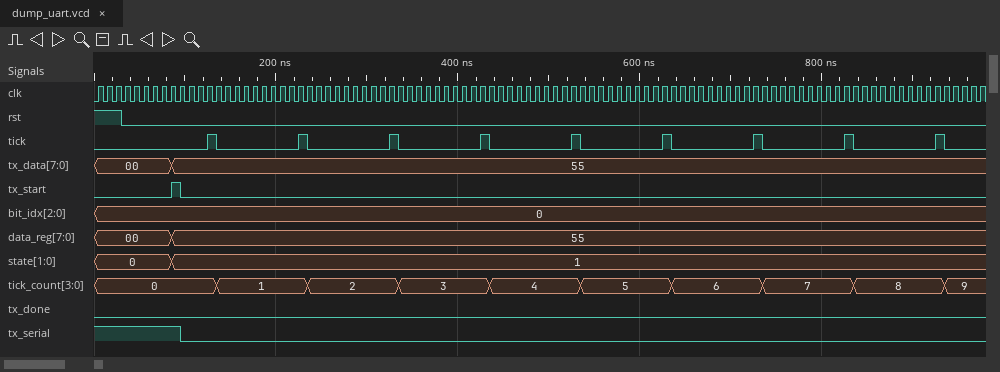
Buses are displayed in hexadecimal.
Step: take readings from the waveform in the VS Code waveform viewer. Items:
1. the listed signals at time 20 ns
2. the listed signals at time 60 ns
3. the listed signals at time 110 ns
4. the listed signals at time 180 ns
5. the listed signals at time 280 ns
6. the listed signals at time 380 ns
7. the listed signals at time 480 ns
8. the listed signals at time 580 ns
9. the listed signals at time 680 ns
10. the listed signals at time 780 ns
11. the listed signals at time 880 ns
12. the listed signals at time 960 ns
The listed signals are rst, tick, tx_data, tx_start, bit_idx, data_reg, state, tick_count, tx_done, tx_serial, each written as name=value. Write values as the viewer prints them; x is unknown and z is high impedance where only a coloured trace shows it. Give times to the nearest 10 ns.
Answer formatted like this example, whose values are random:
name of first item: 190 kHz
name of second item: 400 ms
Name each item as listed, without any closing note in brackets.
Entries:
the listed signals at time 20 ns: rst=1, tick=0, tx_data=00, tx_start=0, bit_idx=0, data_reg=00, state=0, tick_count=0, tx_done=0, tx_serial=1
the listed signals at time 60 ns: rst=0, tick=0, tx_data=00, tx_start=0, bit_idx=0, data_reg=00, state=0, tick_count=0, tx_done=0, tx_serial=1
the listed signals at time 110 ns: rst=0, tick=0, tx_data=55, tx_start=0, bit_idx=0, data_reg=55, state=1, tick_count=0, tx_done=0, tx_serial=0
the listed signals at time 180 ns: rst=0, tick=0, tx_data=55, tx_start=0, bit_idx=0, data_reg=55, state=1, tick_count=1, tx_done=0, tx_serial=0
the listed signals at time 280 ns: rst=0, tick=0, tx_data=55, tx_start=0, bit_idx=0, data_reg=55, state=1, tick_count=2, tx_done=0, tx_serial=0
the listed signals at time 380 ns: rst=0, tick=0, tx_data=55, tx_start=0, bit_idx=0, data_reg=55, state=1, tick_count=3, tx_done=0, tx_serial=0
the listed signals at time 480 ns: rst=0, tick=0, tx_data=55, tx_start=0, bit_idx=0, data_reg=55, state=1, tick_count=4, tx_done=0, tx_serial=0
the listed signals at time 580 ns: rst=0, tick=0, tx_data=55, tx_start=0, bit_idx=0, data_reg=55, state=1, tick_count=5, tx_done=0, tx_serial=0
the listed signals at time 680 ns: rst=0, tick=0, tx_data=55, tx_start=0, bit_idx=0, data_reg=55, state=1, tick_count=6, tx_done=0, tx_serial=0
the listed signals at time 780 ns: rst=0, tick=0, tx_data=55, tx_start=0, bit_idx=0, data_reg=55, state=1, tick_count=7, tx_done=0, tx_serial=0
the listed signals at time 880 ns: rst=0, tick=0, tx_data=55, tx_start=0, bit_idx=0, data_reg=55, state=1, tick_count=8, tx_done=0, tx_serial=0
the listed signals at time 960 ns: rst=0, tick=0, tx_data=55, tx_start=0, bit_idx=0, data_reg=55, state=1, tick_count=9, tx_done=0, tx_serial=0
